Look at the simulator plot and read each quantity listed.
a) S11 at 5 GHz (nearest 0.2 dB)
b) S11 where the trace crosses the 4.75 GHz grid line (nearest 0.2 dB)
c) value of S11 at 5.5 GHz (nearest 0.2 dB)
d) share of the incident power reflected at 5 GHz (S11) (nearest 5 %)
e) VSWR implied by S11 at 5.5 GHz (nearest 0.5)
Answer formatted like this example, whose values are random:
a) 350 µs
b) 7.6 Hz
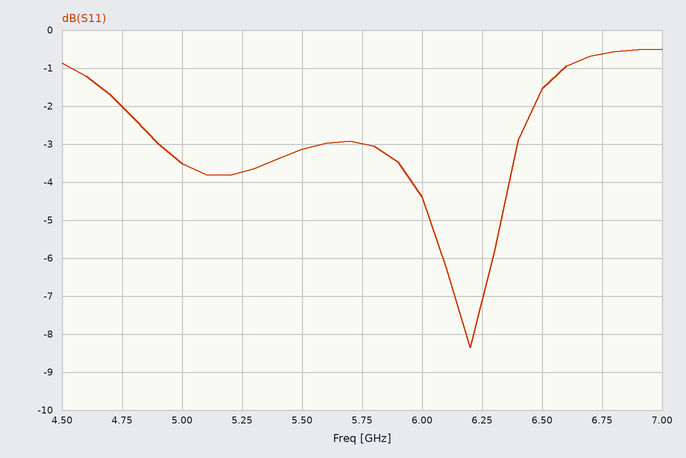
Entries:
a) -3.6 dB
b) -2.0 dB
c) -3.2 dB
d) 45 %
e) 5.5
